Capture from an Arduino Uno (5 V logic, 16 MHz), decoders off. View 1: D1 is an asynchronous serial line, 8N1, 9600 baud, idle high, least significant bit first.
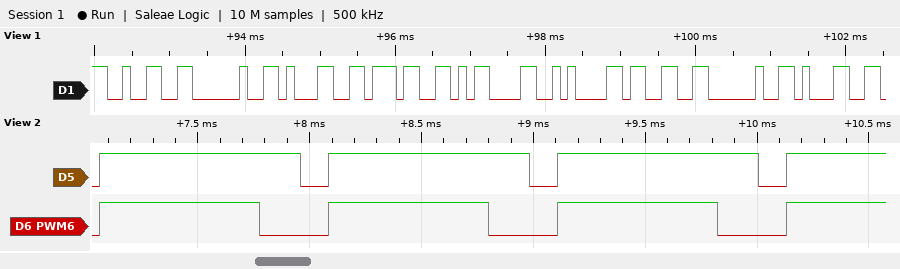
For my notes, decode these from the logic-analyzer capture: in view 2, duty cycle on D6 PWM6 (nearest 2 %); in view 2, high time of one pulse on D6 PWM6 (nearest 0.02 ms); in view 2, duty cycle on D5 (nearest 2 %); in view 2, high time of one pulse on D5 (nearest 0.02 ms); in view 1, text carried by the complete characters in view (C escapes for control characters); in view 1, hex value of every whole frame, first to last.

70 %
0.72 ms
88 %
0.90 ms
"2 17\r\n3 1"
0x32 0x20 0x31 0x37 0x0D 0x0A 0x33 0x20 0x31
